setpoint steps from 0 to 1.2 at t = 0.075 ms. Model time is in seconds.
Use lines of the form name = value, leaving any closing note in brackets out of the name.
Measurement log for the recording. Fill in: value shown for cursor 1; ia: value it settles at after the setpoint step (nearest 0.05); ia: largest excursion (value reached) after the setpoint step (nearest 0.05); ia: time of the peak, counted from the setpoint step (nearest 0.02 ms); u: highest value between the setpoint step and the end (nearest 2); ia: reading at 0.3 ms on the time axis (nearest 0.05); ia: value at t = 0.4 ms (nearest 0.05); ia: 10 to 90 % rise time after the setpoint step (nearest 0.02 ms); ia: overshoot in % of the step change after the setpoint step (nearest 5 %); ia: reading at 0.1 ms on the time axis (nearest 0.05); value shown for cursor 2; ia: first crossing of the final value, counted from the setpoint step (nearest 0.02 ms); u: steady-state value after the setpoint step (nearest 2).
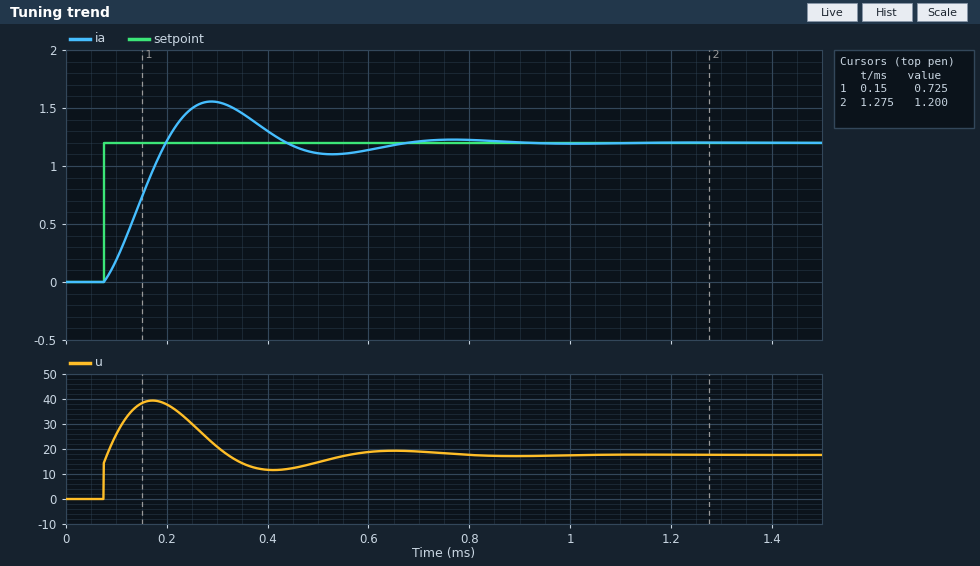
value shown for cursor 1 = 0.725
ia: value it settles at after the setpoint step = 1.20
ia: largest excursion (value reached) after the setpoint step = 1.55
ia: time of the peak, counted from the setpoint step = 0.22 ms
u: highest value between the setpoint step and the end = 40
ia: reading at 0.3 ms on the time axis = 1.55
ia: value at t = 0.4 ms = 1.30
ia: 10 to 90 % rise time after the setpoint step = 0.10 ms
ia: overshoot in % of the step change after the setpoint step = 30 %
ia: reading at 0.1 ms on the time axis = 0.20
value shown for cursor 2 = 1.200
ia: first crossing of the final value, counted from the setpoint step = 0.12 ms
u: steady-state value after the setpoint step = 18
